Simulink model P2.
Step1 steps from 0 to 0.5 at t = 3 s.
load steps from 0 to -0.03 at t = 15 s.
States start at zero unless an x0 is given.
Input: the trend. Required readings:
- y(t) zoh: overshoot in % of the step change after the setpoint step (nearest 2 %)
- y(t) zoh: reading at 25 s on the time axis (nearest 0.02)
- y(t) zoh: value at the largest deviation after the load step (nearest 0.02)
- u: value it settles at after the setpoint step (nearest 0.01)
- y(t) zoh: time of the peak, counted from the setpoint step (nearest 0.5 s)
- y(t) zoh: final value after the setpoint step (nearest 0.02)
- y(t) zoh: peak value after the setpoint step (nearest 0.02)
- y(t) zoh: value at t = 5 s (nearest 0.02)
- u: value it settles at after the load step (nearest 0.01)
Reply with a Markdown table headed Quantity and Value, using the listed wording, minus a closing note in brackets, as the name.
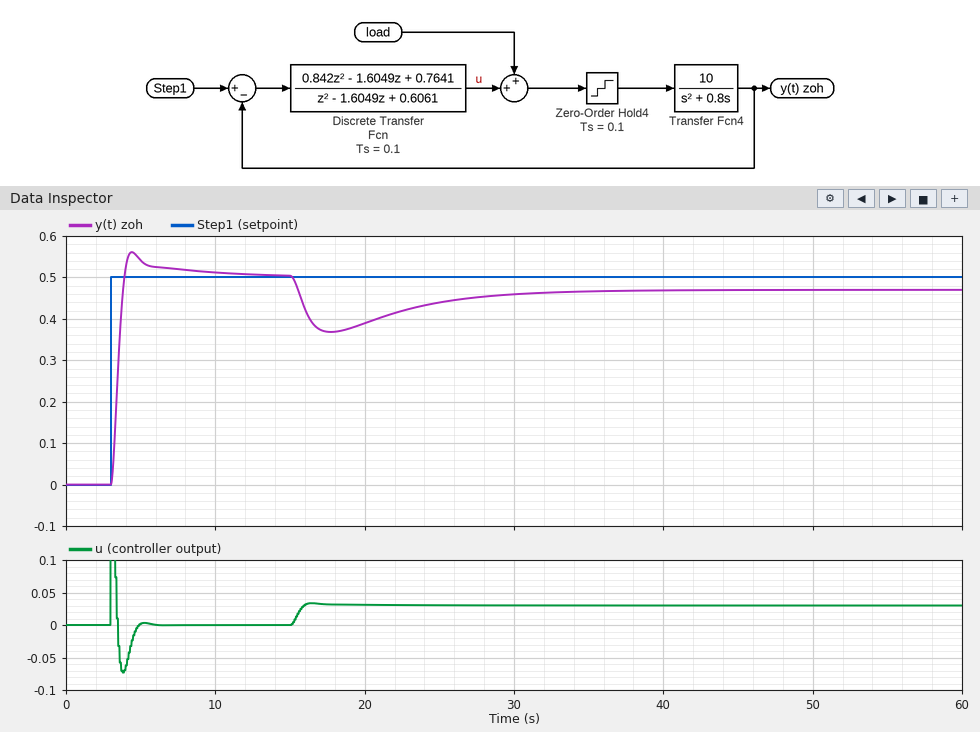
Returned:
| Quantity | Value |
|---|---|
| y(t) zoh: overshoot in % of the step change after the setpoint step | 12 % |
| y(t) zoh: reading at 25 s on the time axis | 0.44 |
| y(t) zoh: value at the largest deviation after the load step | 0.36 |
| u: value it settles at after the setpoint step | 0.00 |
| y(t) zoh: time of the peak, counted from the setpoint step | 1.5 s |
| y(t) zoh: final value after the setpoint step | 0.50 |
| y(t) zoh: peak value after the setpoint step | 0.56 |
| y(t) zoh: value at t = 5 s | 0.54 |
| u: value it settles at after the load step | 0.03 |
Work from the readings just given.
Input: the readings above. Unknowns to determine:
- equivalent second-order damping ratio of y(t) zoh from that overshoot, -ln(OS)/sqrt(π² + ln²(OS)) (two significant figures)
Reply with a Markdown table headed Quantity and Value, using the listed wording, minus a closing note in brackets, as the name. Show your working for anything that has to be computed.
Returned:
| Quantity | Value |
|---|---|
| equivalent second-order damping ratio of y(t) zoh from that overshoot, -ln(OS)/sqrt(π² + ln²(OS)) | ln(0.12) = -2.120; 2.120 / sqrt(9.870 + 4.496) = 0.56 |
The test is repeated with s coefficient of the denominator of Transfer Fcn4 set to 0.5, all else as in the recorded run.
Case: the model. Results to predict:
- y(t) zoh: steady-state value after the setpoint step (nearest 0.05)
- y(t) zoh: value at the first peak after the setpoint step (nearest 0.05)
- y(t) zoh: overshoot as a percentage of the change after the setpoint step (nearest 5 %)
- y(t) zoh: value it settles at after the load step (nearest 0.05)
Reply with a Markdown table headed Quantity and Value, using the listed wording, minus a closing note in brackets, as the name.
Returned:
| Quantity | Value |
|---|---|
| y(t) zoh: steady-state value after the setpoint step | 0.50 |
| y(t) zoh: value at the first peak after the setpoint step | 0.60 |
| y(t) zoh: overshoot as a percentage of the change after the setpoint step | 25 % |
| y(t) zoh: value it settles at after the load step | 0.45 |
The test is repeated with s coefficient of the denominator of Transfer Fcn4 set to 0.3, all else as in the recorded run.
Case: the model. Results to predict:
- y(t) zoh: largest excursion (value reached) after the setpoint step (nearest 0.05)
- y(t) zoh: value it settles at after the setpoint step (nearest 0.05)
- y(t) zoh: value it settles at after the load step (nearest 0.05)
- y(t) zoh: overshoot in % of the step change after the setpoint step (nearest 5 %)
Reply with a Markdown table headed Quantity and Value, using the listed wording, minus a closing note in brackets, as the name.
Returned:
| Quantity | Value |
|---|---|
| y(t) zoh: largest excursion (value reached) after the setpoint step | 0.65 |
| y(t) zoh: value it settles at after the setpoint step | 0.50 |
| y(t) zoh: value it settles at after the load step | 0.45 |
| y(t) zoh: overshoot in % of the step change after the setpoint step | 30 % |
